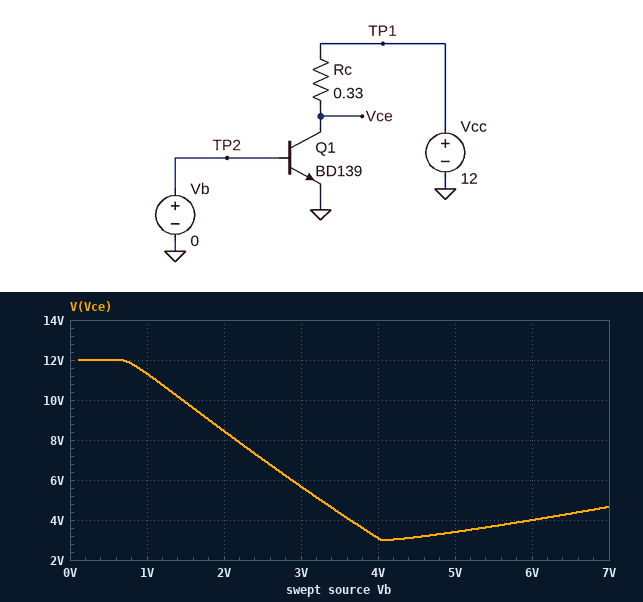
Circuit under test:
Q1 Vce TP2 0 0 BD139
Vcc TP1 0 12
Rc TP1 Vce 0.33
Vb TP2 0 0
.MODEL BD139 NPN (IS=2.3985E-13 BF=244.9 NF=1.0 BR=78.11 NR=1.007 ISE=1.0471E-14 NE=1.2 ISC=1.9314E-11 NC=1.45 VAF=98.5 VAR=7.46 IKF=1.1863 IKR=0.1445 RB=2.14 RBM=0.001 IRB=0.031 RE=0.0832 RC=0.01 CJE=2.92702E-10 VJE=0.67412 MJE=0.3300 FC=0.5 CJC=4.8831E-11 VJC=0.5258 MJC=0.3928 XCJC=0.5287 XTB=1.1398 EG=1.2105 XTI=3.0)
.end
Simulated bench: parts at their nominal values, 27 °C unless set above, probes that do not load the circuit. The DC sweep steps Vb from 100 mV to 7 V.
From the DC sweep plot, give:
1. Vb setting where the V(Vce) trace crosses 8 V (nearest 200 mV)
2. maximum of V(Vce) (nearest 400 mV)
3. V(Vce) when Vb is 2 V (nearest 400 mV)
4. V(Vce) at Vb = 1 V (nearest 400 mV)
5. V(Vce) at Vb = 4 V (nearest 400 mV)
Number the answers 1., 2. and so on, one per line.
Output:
1. 2.2 V
2. 12.0 V
3. 8.4 V
4. 11.2 V
5. 3.2 V
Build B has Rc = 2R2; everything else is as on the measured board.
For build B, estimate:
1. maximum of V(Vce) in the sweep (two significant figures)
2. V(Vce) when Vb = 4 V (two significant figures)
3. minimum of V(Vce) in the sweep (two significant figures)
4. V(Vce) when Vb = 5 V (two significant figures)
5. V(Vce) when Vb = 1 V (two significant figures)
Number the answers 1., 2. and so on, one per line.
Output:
1. 12 V
2. 1.9 V
3. 580 mV
4. 2.6 V
5. 7.5 V
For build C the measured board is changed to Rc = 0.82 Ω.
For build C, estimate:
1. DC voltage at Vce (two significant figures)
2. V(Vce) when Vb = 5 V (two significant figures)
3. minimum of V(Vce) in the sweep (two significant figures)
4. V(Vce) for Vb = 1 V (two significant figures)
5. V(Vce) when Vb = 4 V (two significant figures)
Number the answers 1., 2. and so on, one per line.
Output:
1. 12 V
2. 2.8 V
3. 1.4 V
4. 10 V
5. 2.2 V
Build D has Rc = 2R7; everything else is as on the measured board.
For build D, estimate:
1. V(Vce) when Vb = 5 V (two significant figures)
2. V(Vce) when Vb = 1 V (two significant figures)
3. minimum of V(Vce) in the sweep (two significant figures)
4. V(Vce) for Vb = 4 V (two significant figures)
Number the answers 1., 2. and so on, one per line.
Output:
1. 2.6 V
2. 6.5 V
3. 480 mV
4. 1.9 V
